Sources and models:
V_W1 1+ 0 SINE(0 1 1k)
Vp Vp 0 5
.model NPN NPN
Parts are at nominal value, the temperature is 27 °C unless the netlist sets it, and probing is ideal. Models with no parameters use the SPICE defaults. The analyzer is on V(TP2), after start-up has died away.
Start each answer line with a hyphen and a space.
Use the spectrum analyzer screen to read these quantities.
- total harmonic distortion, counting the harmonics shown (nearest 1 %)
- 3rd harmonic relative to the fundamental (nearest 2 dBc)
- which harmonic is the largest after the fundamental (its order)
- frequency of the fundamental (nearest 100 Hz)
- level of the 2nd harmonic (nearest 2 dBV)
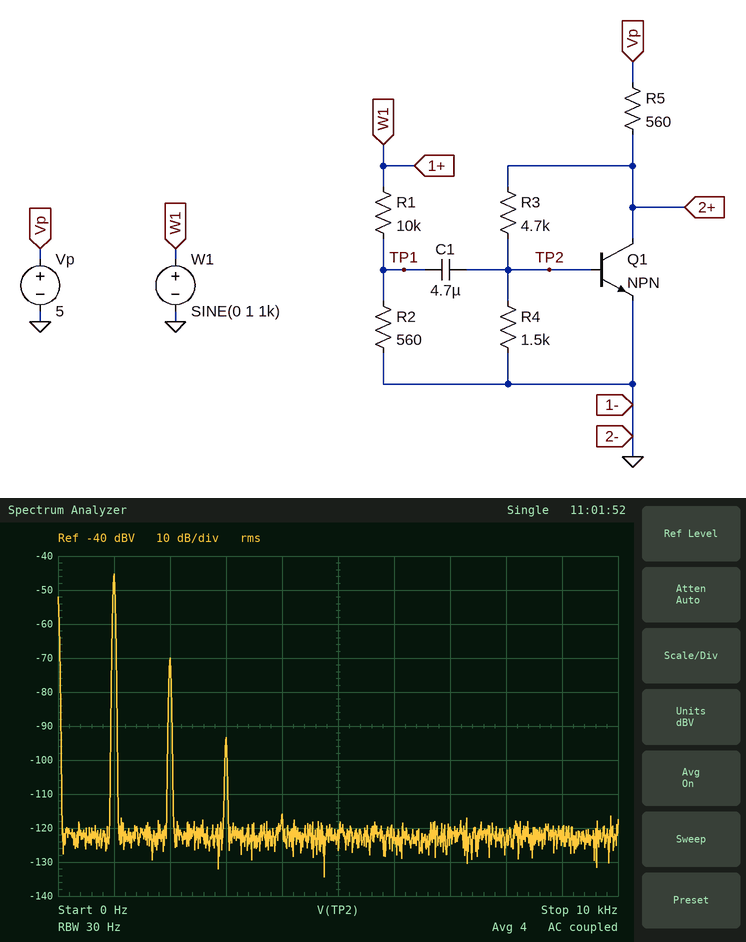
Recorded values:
- 6 %
- -48 dBc
- 2
- 1.0 kHz
- -70 dBV
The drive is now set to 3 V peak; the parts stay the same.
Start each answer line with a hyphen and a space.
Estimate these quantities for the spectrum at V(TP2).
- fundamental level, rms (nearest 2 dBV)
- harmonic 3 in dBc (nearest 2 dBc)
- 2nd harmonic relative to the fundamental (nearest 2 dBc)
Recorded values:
- -34 dBV
- -28 dBc
- -14 dBc
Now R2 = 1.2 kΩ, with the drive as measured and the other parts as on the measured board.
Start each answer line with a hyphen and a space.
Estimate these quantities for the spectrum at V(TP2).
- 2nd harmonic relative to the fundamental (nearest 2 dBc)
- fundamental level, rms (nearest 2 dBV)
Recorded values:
- -24 dBc
- -44 dBV
